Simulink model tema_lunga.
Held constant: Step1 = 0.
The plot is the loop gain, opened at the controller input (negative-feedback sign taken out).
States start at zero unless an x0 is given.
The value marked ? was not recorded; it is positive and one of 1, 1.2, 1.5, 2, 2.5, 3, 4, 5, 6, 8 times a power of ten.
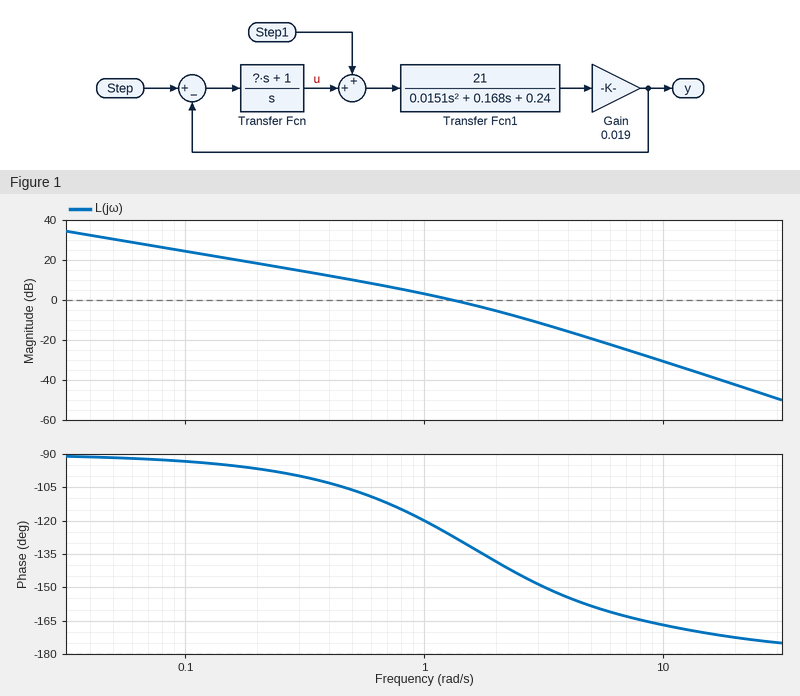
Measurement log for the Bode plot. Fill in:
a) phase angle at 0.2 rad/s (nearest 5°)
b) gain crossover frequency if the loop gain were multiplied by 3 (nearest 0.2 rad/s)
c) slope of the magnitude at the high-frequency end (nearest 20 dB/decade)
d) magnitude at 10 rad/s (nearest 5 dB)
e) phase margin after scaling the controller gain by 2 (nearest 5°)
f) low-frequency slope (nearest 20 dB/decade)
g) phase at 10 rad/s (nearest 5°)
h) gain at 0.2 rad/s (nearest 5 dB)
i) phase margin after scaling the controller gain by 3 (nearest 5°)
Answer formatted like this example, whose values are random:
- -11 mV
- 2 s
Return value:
- -95°
- 2.6 rad/s
- -40 dB/decade
- -30 dB
- 40°
- -20 dB/decade
- -165°
- 20 dB
- 35°
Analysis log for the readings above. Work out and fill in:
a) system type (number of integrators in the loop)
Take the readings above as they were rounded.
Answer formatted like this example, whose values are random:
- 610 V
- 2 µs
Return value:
- 1
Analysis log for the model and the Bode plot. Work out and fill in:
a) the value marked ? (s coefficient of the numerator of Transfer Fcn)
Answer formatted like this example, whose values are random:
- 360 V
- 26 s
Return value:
- 0.12
